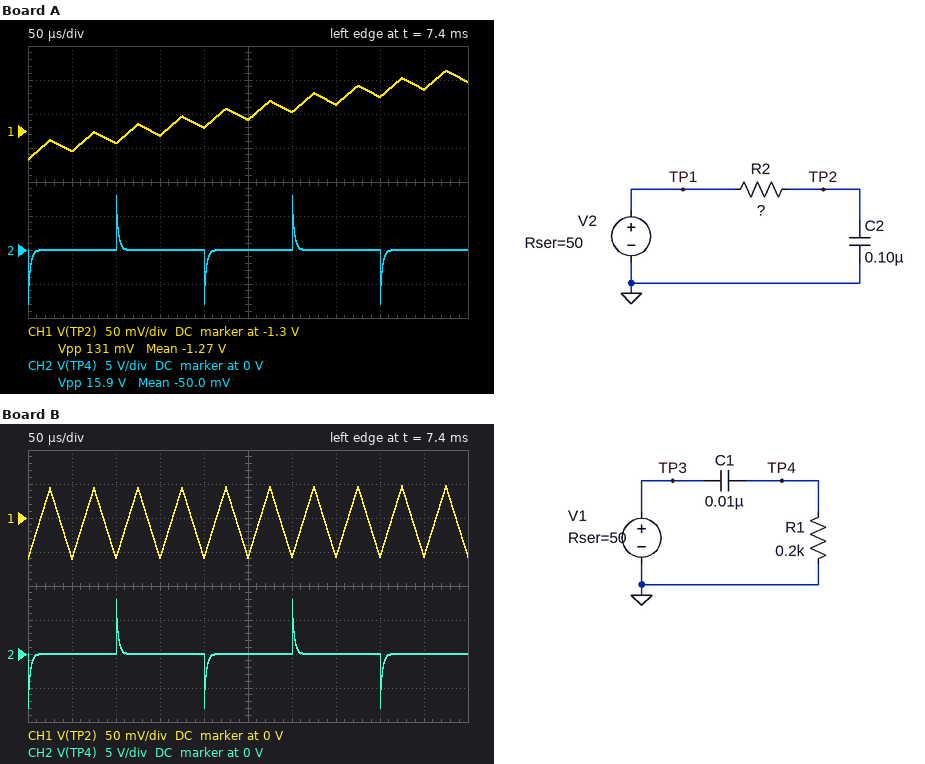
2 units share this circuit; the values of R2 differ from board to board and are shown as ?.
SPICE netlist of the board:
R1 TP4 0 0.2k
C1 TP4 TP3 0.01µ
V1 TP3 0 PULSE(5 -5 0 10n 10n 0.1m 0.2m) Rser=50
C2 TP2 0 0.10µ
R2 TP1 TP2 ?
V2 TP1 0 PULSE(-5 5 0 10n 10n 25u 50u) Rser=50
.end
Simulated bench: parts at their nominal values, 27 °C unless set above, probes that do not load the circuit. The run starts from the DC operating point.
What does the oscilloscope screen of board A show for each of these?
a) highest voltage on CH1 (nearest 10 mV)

-1.21 V
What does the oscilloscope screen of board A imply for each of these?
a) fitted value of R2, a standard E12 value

56 kΩ
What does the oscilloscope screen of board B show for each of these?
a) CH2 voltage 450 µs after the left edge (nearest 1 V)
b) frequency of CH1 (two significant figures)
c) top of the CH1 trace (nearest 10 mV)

0 V
20 kHz
50 mV
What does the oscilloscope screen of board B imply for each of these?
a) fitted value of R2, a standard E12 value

12 kΩ
